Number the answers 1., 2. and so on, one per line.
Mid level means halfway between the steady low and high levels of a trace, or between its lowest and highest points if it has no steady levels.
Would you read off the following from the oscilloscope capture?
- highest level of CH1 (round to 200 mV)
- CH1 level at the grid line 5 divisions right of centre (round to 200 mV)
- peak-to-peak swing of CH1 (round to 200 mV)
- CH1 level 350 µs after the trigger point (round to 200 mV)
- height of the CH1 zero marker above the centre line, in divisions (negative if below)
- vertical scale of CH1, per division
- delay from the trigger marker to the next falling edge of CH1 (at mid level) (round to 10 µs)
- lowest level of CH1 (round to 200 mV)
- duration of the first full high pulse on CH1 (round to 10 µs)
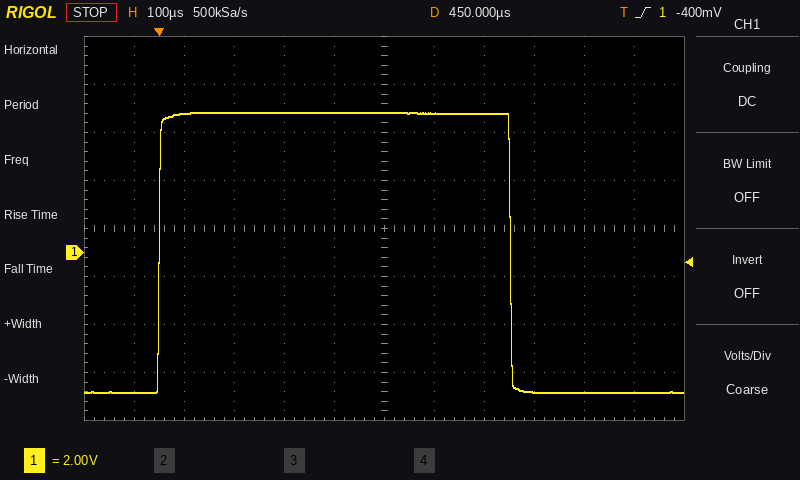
1. 5.8 V
2. -5.8 V
3. 11.6 V
4. 5.8 V
5. -0.5 div
6. 2 V
7. 700 µs
8. -5.8 V
9. 700 µs
